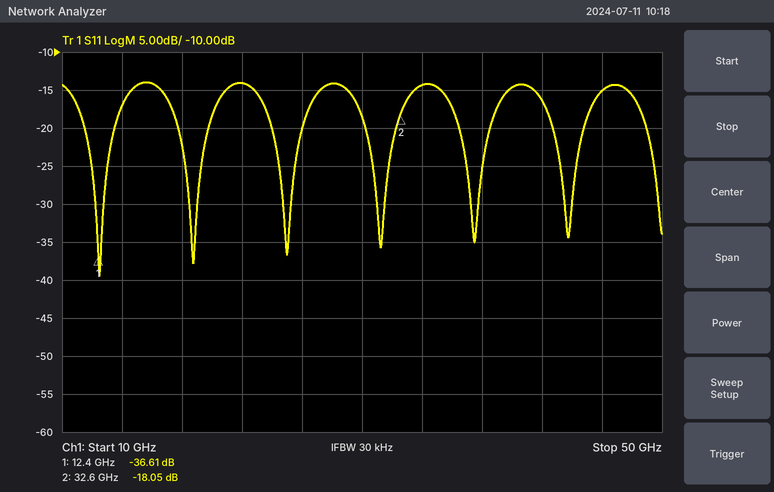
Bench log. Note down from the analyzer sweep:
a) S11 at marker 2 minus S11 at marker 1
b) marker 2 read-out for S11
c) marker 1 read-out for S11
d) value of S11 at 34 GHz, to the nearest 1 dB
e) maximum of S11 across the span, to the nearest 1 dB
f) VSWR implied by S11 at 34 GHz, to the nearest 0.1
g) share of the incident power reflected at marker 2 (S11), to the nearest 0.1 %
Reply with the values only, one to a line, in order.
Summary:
18.56 dB
-18.05 dB
-36.61 dB
-14 dB
-14 dB
1.5
1.6 %
